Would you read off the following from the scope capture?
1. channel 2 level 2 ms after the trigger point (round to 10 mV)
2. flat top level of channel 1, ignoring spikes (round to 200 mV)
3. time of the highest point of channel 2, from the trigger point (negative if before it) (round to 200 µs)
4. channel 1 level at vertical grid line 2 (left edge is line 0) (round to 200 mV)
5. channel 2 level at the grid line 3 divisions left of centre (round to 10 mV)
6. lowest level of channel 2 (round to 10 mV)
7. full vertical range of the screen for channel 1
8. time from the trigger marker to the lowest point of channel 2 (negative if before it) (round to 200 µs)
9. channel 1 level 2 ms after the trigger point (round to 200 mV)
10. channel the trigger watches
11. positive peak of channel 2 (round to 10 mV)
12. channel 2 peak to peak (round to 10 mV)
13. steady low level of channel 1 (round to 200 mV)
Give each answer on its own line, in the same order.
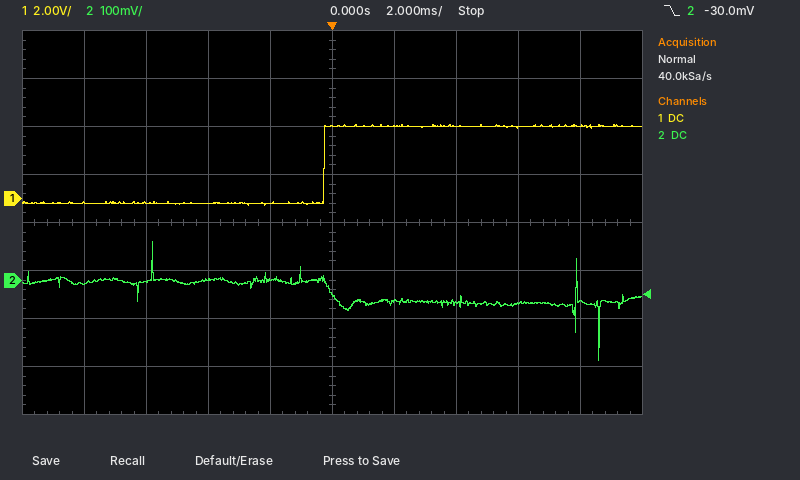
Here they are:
-40 mV
3.0 V
-5.8 ms
-200 mV
0 mV
-170 mV
16 V
+8.6 ms
3.0 V
channel 2
80 mV
250 mV
-200 mV
